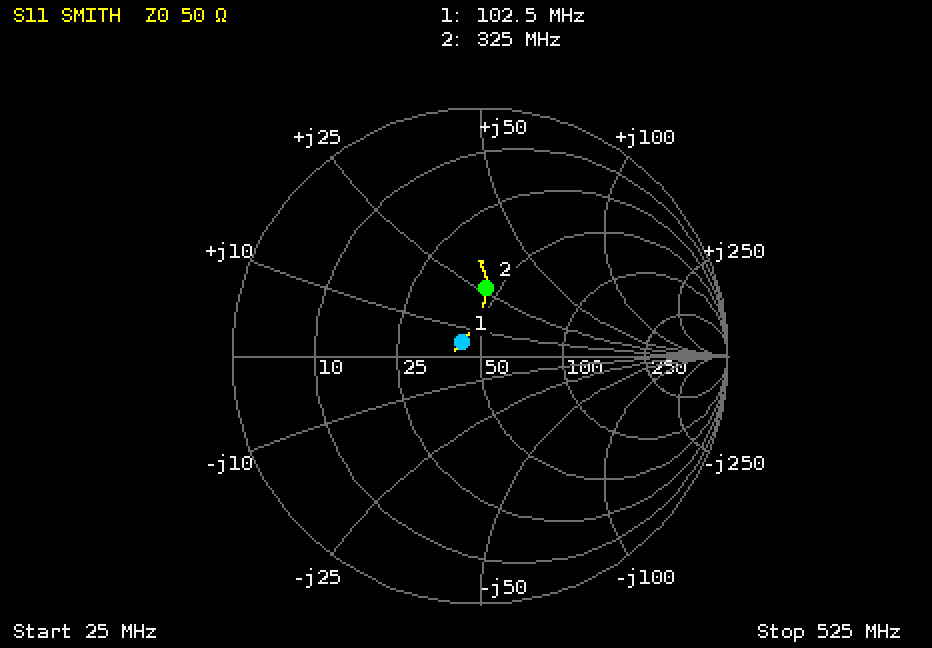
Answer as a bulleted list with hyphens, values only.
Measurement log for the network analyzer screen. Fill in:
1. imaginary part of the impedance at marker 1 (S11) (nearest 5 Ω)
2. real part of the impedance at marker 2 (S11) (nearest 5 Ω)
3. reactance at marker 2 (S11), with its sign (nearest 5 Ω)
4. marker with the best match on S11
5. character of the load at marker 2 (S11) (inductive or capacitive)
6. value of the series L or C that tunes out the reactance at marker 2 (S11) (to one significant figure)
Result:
- +5 Ω
- 45 Ω
- +25 Ω
- marker 1
- inductive
- 20 pF
